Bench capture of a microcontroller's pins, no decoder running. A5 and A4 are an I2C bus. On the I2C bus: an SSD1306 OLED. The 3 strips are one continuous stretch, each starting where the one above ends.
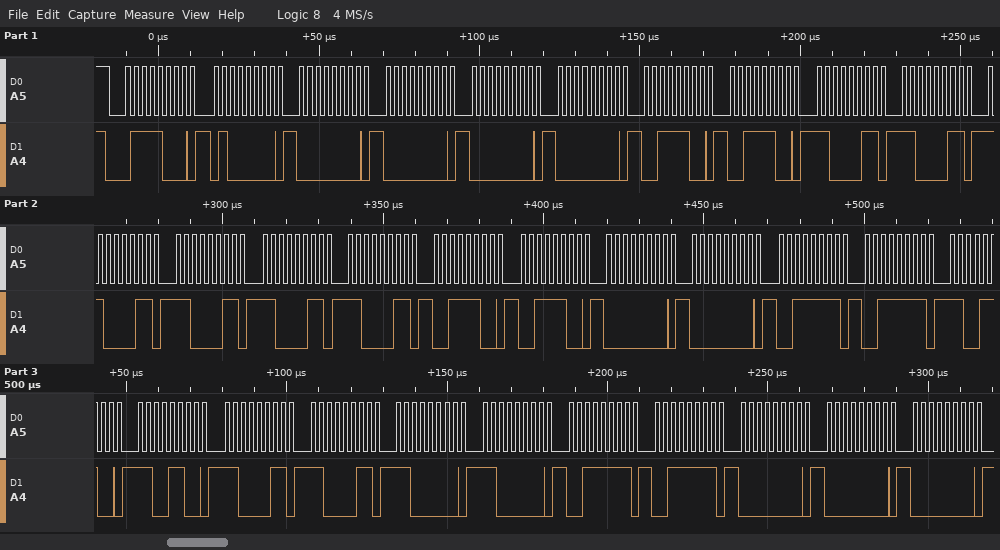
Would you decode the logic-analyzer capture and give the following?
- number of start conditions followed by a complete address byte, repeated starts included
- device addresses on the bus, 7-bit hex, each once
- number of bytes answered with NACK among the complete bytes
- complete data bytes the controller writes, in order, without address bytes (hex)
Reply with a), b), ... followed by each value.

a) 1
b) 0x3C
c) 0
d) 40 00 00 00 00 3C 3C C3 C3 C3 C3 C3 C3 3C 3C 00 00 3F 3F CC CC C3 C3 C0 C0 3F 3F 00 00 00
